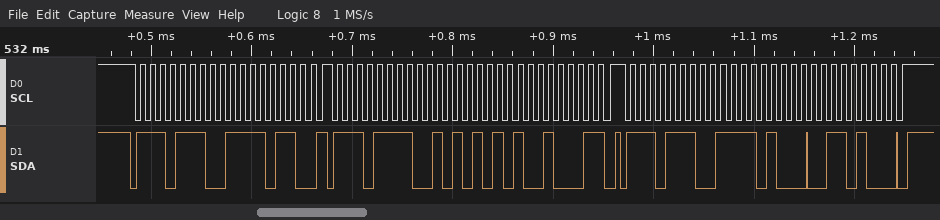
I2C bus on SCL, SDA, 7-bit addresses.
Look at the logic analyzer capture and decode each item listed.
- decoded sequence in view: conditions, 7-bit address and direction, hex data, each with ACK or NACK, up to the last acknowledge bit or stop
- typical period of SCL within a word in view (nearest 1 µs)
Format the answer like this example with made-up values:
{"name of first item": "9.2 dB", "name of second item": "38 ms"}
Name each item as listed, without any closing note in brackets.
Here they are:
{"decoded sequence in view: conditions, 7-bit address and direction, hex data, each with ACK or NACK, up to the last acknowledge bit or stop": "start, address 77 write ACK, F6 ACK, repeated start, address 77 read ACK, 55 ACK, 91 NACK, stop, start, address 77 write ACK, F4 ACK, 34 ACK, stop", "typical period of SCL within a word in view": "10 µs"}
